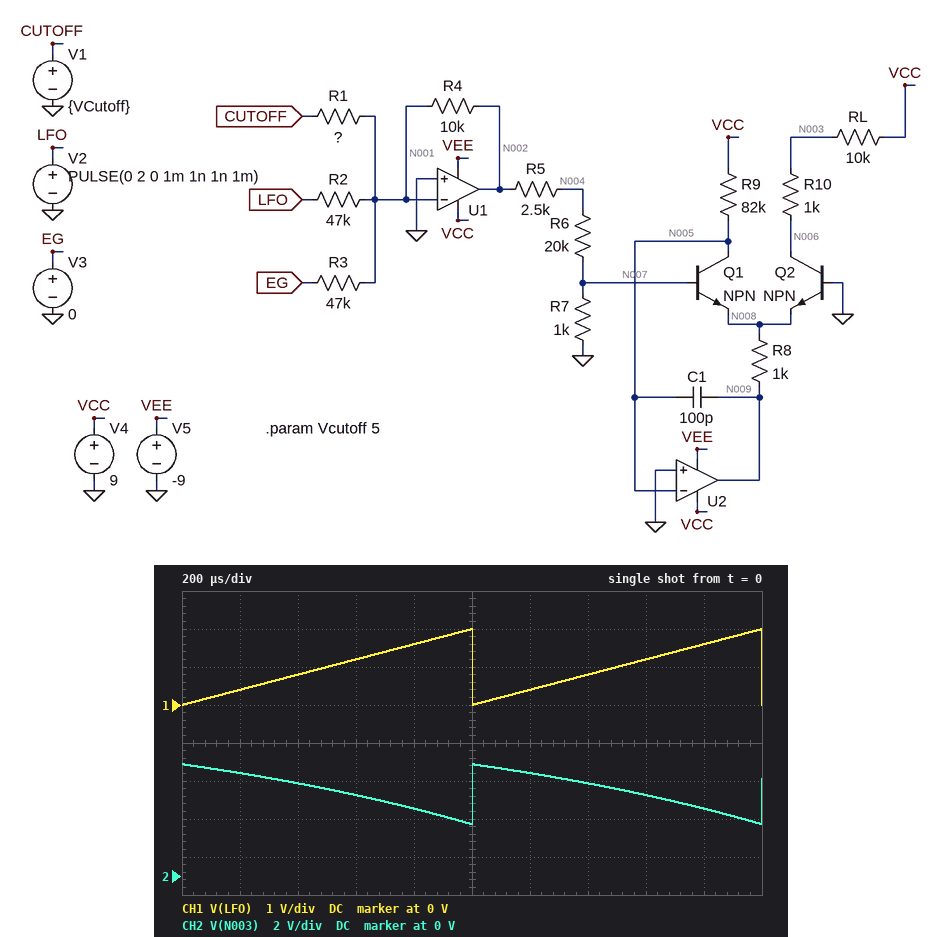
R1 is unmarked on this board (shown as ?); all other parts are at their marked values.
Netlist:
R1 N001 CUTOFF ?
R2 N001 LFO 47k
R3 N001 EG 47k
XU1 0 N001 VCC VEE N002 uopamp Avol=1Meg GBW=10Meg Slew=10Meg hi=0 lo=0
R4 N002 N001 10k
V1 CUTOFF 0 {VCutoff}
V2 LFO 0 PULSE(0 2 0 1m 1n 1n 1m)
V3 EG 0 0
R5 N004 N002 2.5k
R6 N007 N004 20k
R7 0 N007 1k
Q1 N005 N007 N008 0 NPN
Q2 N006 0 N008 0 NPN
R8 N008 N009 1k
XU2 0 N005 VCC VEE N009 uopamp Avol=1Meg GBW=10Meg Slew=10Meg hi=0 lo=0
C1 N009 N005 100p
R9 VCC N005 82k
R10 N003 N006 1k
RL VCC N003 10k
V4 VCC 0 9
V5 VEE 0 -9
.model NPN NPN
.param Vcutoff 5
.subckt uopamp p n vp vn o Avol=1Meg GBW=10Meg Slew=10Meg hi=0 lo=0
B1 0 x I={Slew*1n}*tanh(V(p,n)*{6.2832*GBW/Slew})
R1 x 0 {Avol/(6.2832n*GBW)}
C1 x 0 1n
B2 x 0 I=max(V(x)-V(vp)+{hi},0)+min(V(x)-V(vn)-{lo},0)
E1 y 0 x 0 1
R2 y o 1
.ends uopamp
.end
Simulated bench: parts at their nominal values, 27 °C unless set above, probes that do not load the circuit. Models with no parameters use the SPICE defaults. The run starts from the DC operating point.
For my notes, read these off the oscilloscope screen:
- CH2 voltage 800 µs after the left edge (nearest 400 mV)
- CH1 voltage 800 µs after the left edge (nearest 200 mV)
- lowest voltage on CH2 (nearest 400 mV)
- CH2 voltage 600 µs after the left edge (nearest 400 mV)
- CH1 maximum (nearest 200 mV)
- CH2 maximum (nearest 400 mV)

3.6 V
1.6 V
2.8 V
4.4 V
2.0 V
6.0 V
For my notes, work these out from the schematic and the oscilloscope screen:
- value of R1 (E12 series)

82 kΩ
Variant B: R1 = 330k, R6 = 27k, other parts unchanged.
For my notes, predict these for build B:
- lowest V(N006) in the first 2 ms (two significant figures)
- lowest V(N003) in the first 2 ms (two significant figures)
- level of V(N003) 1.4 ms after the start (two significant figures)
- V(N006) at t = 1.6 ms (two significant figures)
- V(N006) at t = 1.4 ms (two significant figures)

6.4 V
6.6 V
7.3 V
6.9 V
7.1 V
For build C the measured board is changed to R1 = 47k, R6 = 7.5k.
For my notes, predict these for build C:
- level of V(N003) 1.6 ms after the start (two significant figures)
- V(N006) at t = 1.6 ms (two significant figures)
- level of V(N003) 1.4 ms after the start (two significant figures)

75 mV
-820 mV
82 mV
